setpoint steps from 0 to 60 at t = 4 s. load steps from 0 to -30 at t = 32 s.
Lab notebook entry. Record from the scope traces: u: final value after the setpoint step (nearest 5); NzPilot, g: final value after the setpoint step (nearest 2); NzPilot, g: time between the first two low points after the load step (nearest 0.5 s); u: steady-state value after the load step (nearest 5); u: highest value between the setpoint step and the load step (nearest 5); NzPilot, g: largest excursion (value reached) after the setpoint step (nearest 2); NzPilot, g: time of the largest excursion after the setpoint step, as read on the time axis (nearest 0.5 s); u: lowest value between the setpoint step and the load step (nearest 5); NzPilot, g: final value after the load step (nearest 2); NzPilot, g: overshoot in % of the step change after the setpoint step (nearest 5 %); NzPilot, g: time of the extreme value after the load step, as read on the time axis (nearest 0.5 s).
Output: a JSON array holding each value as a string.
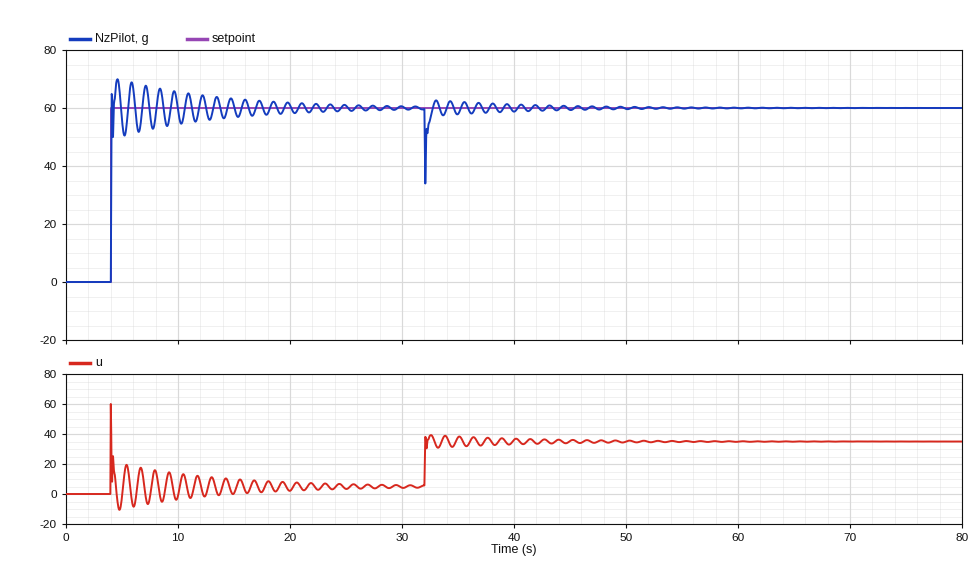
["5", "60", "1.5 s", "35", "60", "70", "4.5 s", "-10", "60", "15 %", "32.0 s"]
